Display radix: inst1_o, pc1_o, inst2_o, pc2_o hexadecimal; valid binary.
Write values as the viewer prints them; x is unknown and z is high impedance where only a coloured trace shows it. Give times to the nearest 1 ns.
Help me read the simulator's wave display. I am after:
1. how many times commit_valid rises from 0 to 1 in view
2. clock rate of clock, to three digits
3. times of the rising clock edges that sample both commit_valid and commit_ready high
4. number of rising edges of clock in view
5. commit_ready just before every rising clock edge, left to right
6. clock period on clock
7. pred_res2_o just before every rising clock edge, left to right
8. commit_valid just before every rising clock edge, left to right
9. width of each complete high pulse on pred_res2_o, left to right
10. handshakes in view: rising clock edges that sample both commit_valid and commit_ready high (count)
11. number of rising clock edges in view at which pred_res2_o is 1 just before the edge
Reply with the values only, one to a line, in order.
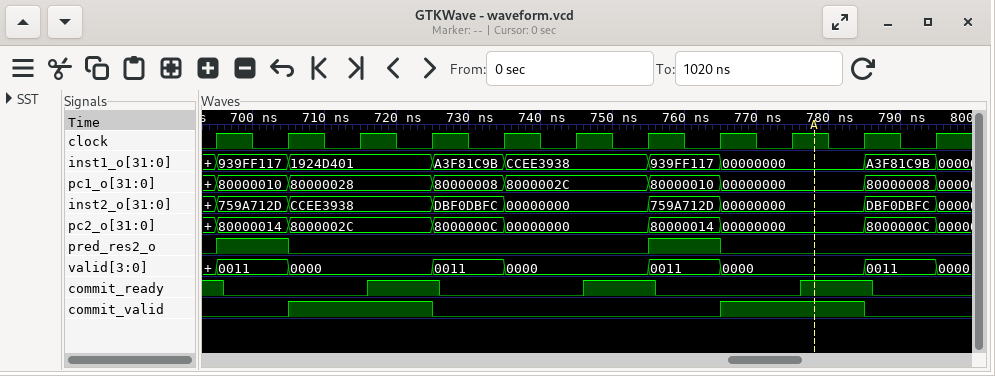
2
100 MHz
725 ns, 785 ns
11
1 0 0 1 0 0 1 0 0 1 0
10 ns
0 1 0 0 0 0 0 1 0 0 0
0 0 1 1 0 0 0 0 1 1 0
10 ns, 10 ns
2
2
